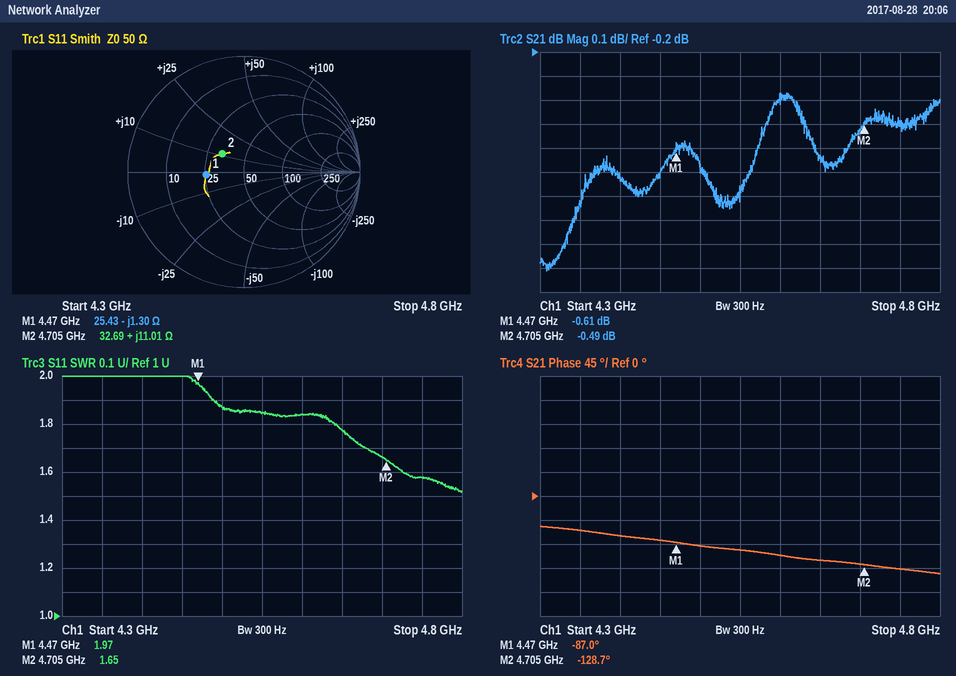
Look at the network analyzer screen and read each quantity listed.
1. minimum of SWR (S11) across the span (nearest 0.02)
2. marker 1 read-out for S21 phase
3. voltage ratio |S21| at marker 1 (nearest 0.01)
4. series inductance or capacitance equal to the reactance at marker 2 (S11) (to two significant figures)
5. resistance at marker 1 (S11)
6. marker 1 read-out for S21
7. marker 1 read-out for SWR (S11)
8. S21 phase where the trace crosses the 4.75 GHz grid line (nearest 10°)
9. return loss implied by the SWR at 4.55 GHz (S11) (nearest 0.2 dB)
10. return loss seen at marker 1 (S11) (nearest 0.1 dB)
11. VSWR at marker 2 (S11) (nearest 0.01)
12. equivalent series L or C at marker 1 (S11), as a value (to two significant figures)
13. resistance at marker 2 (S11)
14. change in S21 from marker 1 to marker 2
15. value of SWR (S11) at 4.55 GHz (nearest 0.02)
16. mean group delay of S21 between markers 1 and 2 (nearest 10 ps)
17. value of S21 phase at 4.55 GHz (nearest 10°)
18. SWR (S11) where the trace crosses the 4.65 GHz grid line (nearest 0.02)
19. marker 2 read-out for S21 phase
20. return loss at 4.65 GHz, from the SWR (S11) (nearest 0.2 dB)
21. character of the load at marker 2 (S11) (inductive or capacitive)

1.52
-87.0°
0.93
370 pH
25.43 Ω
-0.61 dB
1.97
-140°
10.6 dB
9.7 dB
1.65
27 pF
32.69 Ω
0.12 dB
1.84
490 ps
-100°
1.78
-128.7°
11.0 dB
inductive
